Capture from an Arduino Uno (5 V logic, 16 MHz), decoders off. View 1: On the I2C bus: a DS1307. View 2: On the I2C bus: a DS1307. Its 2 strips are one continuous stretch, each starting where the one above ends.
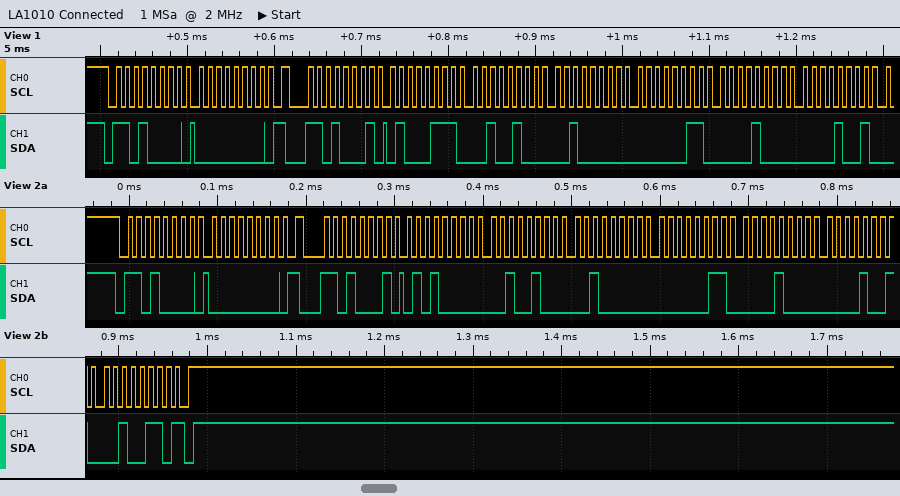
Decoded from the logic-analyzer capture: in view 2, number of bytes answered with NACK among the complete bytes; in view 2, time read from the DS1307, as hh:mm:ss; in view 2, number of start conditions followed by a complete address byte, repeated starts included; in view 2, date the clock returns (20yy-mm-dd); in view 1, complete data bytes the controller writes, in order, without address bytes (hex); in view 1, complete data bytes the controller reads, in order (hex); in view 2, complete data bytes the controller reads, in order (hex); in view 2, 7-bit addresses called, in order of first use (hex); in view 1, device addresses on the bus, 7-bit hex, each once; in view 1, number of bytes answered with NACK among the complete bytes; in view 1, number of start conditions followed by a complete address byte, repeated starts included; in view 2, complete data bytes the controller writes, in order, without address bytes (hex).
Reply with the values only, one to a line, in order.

1
20:24:50
2
2026-09-08
00
47 24 20 03 08 09
50 24 20 03 08 09 26
0x68
0x68
0
2
00
